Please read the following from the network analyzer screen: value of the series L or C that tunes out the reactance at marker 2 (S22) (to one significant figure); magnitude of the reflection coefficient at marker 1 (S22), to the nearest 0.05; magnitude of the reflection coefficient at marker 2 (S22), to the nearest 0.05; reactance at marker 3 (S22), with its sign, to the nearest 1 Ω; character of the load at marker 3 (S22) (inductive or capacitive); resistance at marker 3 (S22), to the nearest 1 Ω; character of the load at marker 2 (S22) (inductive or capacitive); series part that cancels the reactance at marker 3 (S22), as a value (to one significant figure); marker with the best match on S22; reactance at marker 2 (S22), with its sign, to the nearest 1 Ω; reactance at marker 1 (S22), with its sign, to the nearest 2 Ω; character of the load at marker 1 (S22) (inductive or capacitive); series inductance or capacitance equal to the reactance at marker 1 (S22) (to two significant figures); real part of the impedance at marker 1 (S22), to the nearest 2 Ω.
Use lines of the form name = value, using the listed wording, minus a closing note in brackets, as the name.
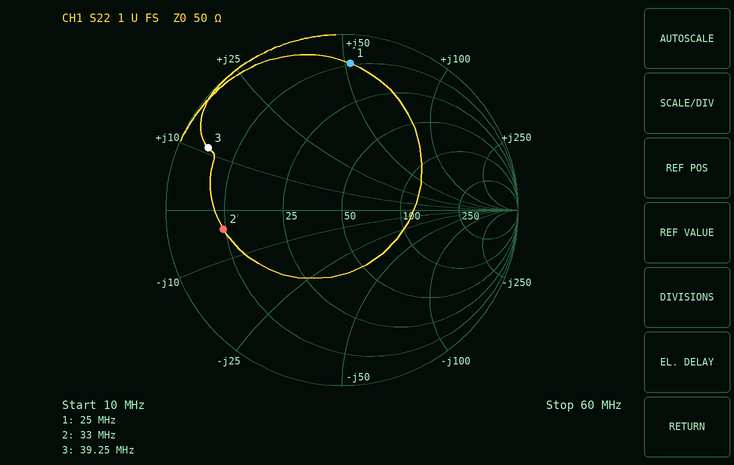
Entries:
value of the series L or C that tunes out the reactance at marker 2 (S22) = 20 nH
magnitude of the reflection coefficient at marker 1 (S22), to the nearest 0.05 = 0.85
magnitude of the reflection coefficient at marker 2 (S22), to the nearest 0.05 = 0.70
reactance at marker 3 (S22), with its sign, to the nearest 1 Ω = +11 Ω
character of the load at marker 3 (S22) = inductive
resistance at marker 3 (S22), to the nearest 1 Ω = 5 Ω
character of the load at marker 2 (S22) = capacitive
series part that cancels the reactance at marker 3 (S22), as a value = 400 pF
marker with the best match on S22 = marker 2
reactance at marker 2 (S22), with its sign, to the nearest 1 Ω = -4 Ω
reactance at marker 1 (S22), with its sign, to the nearest 2 Ω = +52 Ω
character of the load at marker 1 (S22) = inductive
series inductance or capacitance equal to the reactance at marker 1 (S22) = 330 nH
real part of the impedance at marker 1 (S22), to the nearest 2 Ω = 10 Ω
